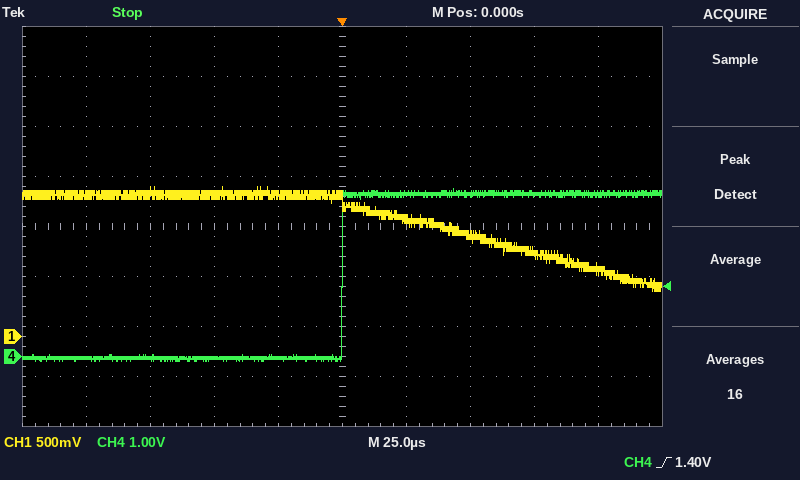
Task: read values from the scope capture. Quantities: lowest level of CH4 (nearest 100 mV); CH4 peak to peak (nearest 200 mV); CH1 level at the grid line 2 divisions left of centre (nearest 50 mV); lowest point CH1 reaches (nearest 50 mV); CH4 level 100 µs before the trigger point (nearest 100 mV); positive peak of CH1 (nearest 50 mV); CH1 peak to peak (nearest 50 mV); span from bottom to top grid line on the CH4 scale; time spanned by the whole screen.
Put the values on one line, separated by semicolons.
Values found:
-100 mV; 3.4 V; 1.40 V; 450 mV; 0.0 V; 1.50 V; 1.05 V; 8 V; 250 µs
